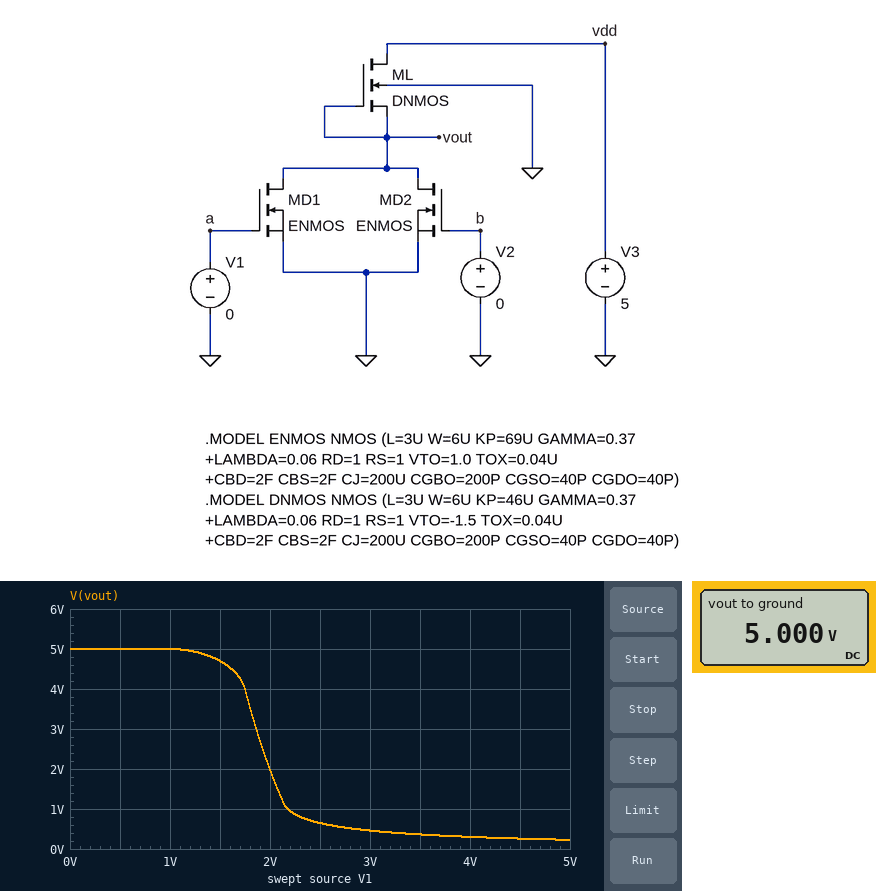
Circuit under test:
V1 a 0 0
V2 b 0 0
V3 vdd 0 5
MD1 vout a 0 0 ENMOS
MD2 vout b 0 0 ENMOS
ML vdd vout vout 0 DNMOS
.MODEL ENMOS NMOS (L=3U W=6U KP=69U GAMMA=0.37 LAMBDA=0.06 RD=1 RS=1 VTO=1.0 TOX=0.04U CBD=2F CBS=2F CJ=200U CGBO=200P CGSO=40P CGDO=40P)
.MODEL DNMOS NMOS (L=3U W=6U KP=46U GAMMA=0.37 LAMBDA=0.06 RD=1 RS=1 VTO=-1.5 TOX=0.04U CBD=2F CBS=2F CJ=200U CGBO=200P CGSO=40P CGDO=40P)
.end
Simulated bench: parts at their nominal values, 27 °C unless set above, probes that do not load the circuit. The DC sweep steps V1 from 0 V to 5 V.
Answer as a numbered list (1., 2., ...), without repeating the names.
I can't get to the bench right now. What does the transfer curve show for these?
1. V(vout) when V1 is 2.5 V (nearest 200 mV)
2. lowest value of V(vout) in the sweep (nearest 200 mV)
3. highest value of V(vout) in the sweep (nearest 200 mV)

1. 600 mV
2. 200 mV
3. 5.0 V
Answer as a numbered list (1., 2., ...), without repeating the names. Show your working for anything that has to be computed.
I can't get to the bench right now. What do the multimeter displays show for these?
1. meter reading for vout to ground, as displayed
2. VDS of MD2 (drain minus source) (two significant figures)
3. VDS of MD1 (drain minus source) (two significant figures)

1. 5.000 V
2. 5 V = 5.0 V
3. 5 V = 5.0 V
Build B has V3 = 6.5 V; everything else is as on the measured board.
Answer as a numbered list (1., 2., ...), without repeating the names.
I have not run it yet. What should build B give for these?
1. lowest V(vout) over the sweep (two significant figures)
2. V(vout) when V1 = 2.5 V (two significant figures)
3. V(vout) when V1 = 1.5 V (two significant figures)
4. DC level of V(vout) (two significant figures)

1. 240 mV
2. 700 mV
3. 6.1 V
4. 6.5 V
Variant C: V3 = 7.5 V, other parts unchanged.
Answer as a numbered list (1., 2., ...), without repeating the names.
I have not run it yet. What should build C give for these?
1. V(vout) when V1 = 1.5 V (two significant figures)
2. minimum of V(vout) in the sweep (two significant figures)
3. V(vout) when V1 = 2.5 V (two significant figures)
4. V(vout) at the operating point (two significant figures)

1. 7.0 V
2. 250 mV
3. 730 mV
4. 7.5 V
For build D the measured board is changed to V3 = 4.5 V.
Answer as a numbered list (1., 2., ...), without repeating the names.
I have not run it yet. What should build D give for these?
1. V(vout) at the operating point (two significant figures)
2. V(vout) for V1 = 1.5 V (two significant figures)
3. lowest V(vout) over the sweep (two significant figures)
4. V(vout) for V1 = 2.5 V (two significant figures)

1. 4.5 V
2. 4.2 V
3. 220 mV
4. 630 mV
